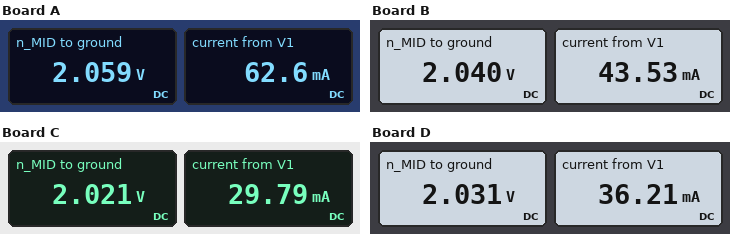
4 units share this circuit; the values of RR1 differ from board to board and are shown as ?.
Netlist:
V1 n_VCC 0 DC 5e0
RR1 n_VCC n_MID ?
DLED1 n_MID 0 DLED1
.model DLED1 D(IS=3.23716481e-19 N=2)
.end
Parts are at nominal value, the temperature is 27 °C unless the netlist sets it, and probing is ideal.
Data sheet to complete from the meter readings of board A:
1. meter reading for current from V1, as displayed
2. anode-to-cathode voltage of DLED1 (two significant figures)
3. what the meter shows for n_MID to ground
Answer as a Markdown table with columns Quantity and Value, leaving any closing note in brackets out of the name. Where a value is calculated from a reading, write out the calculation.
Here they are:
| Quantity | Value |
|---|---|
| meter reading for current from V1, as displayed | 62.6 mA |
| anode-to-cathode voltage of DLED1 | 2.059 V = 2.1 V |
| what the meter shows for n_MID to ground | 2.059 V |
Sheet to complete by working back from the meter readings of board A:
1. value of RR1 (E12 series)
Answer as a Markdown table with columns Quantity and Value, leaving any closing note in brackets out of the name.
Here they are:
| Quantity | Value |
|---|---|
| value of RR1 | 47 Ω |
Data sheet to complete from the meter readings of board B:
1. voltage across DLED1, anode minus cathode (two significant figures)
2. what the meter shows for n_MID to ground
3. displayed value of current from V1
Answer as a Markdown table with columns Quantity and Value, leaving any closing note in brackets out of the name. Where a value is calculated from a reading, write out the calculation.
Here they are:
| Quantity | Value |
|---|---|
| voltage across DLED1, anode minus cathode | 2.04 V = 2.0 V |
| what the meter shows for n_MID to ground | 2.040 V |
| displayed value of current from V1 | 43.53 mA |
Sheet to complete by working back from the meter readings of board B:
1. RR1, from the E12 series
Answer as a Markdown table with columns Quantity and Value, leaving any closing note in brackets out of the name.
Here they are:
| Quantity | Value |
|---|---|
| RR1, from the E12 series | 68 Ω |
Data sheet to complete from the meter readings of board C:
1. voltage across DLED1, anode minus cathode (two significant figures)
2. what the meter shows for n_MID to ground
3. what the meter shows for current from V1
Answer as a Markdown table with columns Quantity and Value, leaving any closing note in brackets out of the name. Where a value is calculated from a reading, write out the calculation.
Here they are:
| Quantity | Value |
|---|---|
| voltage across DLED1, anode minus cathode | 2.021 V = 2.0 V |
| what the meter shows for n_MID to ground | 2.021 V |
| what the meter shows for current from V1 | 29.79 mA |
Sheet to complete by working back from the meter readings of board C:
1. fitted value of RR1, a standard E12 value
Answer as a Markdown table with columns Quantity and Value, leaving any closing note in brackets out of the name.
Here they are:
| Quantity | Value |
|---|---|
| fitted value of RR1, a standard E12 value | 100 Ω |
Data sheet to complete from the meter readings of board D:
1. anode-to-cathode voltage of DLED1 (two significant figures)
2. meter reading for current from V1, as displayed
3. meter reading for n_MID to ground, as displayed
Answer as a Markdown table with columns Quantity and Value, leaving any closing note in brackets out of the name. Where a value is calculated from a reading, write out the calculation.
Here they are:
| Quantity | Value |
|---|---|
| anode-to-cathode voltage of DLED1 | 2.031 V = 2.0 V |
| meter reading for current from V1, as displayed | 36.21 mA |
| meter reading for n_MID to ground, as displayed | 2.031 V |
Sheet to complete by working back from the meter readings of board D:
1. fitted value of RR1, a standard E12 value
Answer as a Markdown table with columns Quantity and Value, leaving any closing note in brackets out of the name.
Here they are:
| Quantity | Value |
|---|---|
| fitted value of RR1, a standard E12 value | 82 Ω |
